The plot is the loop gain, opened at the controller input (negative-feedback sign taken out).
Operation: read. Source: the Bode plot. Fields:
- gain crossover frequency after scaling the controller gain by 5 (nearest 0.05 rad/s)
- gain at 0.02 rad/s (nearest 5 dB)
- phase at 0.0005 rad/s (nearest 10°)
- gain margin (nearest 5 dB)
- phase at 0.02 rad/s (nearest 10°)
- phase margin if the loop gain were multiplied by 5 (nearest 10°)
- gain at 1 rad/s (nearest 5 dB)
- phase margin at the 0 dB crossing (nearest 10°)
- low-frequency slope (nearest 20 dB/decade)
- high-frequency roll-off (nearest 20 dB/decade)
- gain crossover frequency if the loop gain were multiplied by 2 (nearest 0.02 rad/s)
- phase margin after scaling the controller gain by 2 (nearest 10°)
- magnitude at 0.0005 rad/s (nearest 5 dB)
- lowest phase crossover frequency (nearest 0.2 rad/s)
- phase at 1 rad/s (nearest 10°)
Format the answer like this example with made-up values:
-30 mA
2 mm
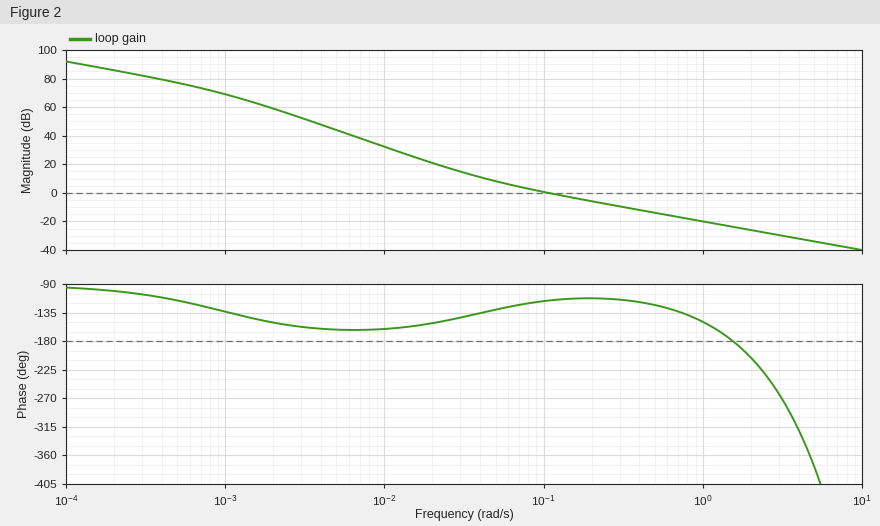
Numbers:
0.50 rad/s
20 dB
-120°
25 dB
-150°
60°
-20 dB
60°
-20 dB/decade
-20 dB/decade
0.20 rad/s
70°
75 dB
1.6 rad/s
-150°
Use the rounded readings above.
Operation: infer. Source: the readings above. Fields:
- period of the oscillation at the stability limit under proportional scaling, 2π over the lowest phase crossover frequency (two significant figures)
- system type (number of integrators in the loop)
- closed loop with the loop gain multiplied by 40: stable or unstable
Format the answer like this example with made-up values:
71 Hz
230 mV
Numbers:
3.9 s
1
unstable
